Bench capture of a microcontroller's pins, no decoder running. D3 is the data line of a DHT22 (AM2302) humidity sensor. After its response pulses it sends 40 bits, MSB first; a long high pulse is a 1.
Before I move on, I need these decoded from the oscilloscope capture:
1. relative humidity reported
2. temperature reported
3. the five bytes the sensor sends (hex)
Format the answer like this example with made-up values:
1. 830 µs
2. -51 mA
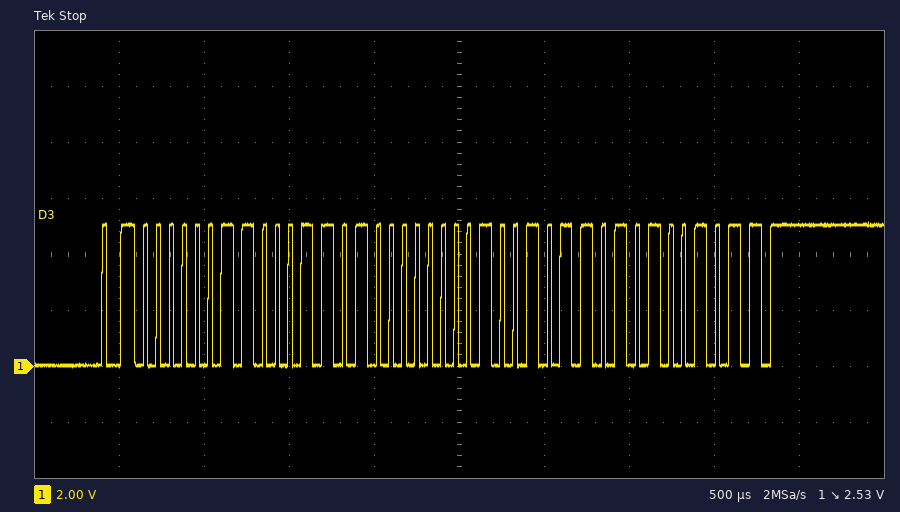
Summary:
1. 79.4 %
2. 30.1 °C
3. 03 1A 01 2D 4B
